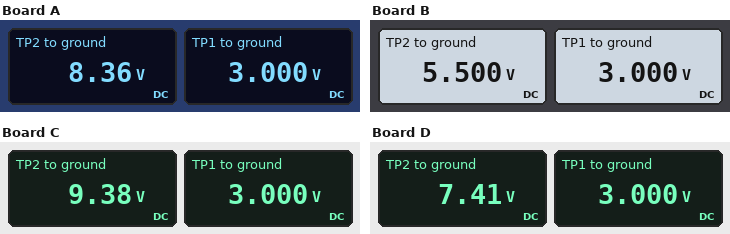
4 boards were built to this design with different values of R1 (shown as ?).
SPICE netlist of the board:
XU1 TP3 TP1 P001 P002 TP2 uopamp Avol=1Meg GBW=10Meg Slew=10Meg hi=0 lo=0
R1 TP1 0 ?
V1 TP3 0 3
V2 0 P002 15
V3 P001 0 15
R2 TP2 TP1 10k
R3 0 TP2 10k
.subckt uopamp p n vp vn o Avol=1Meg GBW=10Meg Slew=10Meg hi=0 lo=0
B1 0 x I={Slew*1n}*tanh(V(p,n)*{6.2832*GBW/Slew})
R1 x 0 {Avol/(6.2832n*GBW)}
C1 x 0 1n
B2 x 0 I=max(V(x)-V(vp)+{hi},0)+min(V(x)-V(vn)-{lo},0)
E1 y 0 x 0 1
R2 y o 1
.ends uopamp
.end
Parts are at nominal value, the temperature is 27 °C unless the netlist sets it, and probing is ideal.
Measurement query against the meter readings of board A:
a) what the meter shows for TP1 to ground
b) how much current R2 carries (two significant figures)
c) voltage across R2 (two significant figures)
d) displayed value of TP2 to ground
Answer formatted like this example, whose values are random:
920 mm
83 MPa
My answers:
3.000 V
540 µA
5.4 V
8.36 V
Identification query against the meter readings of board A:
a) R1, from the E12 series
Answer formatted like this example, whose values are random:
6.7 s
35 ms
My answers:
5.6 kΩ
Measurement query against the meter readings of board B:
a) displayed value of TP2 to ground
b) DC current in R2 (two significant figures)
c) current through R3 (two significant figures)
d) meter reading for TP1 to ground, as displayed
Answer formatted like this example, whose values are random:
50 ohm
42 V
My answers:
5.500 V
250 µA
550 µA
3.000 V
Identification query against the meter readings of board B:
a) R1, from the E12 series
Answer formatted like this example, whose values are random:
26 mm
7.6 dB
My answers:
12 kΩ
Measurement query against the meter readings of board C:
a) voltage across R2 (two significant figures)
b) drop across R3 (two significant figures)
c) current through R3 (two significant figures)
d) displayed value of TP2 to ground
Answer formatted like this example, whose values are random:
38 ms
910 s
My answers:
6.4 V
9.4 V
940 µA
9.38 V
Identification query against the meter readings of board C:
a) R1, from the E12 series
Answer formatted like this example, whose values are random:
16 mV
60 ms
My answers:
4.7 kΩ
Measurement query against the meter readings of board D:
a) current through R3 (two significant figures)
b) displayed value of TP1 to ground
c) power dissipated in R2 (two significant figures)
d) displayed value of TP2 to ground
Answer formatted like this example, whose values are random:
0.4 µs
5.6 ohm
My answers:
740 µA
3.000 V
1.9 mW
7.41 V
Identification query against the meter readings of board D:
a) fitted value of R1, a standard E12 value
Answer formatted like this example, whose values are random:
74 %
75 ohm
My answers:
6.8 kΩ
